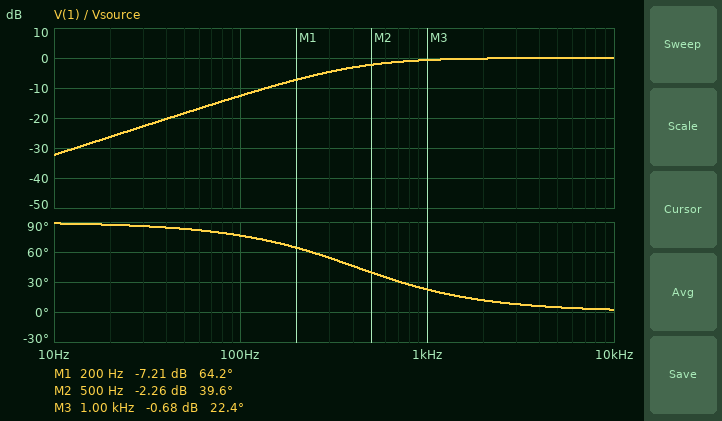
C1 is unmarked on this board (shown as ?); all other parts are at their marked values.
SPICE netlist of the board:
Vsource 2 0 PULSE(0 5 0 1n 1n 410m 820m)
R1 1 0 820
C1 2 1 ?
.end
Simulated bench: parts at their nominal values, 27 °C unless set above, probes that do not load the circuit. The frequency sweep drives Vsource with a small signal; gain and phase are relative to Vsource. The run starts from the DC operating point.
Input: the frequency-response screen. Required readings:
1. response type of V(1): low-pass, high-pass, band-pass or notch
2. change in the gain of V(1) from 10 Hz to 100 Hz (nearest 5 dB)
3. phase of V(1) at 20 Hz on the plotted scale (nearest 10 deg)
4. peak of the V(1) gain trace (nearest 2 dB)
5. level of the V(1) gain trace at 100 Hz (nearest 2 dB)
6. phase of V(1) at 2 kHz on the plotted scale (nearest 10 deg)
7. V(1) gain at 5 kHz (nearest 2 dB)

high-pass
20 dB
90 deg
0 dB
-12 dB
10 deg
0 dB
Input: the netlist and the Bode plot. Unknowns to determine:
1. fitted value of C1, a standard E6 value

470 nF
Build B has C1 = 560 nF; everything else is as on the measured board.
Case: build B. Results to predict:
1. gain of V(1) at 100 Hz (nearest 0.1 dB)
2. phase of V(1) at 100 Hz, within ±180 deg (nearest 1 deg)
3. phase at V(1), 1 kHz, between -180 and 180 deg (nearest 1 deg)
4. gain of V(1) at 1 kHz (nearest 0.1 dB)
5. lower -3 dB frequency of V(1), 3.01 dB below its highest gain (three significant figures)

-11.1 dB
74 deg
19 deg
-0.5 dB
347 Hz
